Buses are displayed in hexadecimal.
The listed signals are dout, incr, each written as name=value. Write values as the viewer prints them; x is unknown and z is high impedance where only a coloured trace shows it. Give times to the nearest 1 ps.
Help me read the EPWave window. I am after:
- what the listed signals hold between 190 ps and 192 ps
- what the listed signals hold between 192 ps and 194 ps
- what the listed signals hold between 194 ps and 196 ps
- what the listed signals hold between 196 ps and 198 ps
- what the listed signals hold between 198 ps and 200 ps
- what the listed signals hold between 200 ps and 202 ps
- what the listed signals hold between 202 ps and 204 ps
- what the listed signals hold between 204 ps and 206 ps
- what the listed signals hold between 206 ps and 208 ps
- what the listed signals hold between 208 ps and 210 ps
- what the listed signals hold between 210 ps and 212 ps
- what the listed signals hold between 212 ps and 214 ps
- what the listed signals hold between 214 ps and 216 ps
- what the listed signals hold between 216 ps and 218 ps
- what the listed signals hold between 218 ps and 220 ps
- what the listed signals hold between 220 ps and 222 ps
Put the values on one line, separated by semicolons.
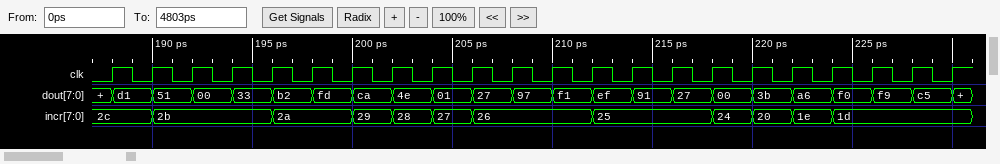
dout=51, incr=2b; dout=00, incr=2b; dout=33, incr=2b; dout=b2, incr=2a; dout=fd, incr=2a; dout=ca, incr=29; dout=4e, incr=28; dout=01, incr=27; dout=27, incr=26; dout=97, incr=26; dout=f1, incr=26; dout=ef, incr=25; dout=91, incr=25; dout=27, incr=25; dout=00, incr=24; dout=3b, incr=20
